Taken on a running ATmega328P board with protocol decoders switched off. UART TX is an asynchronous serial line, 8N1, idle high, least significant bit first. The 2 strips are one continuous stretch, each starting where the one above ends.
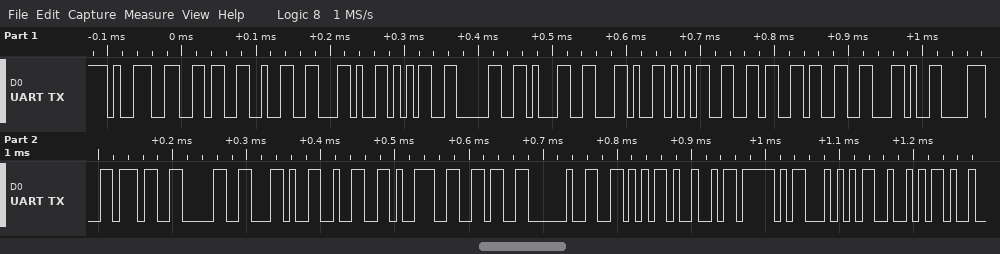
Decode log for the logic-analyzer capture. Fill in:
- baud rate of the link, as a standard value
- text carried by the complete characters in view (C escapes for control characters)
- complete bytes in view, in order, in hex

115200 baud
"962,501,563,870,296 VI_TR"
0x39 0x36 0x32 0x2C 0x35 0x30 0x31 0x2C 0x35 0x36 0x33 0x2C 0x38 0x37 0x30 0x2C 0x32 0x39 0x36 0x20 0x56 0x49 0x5F 0x54 0x52
